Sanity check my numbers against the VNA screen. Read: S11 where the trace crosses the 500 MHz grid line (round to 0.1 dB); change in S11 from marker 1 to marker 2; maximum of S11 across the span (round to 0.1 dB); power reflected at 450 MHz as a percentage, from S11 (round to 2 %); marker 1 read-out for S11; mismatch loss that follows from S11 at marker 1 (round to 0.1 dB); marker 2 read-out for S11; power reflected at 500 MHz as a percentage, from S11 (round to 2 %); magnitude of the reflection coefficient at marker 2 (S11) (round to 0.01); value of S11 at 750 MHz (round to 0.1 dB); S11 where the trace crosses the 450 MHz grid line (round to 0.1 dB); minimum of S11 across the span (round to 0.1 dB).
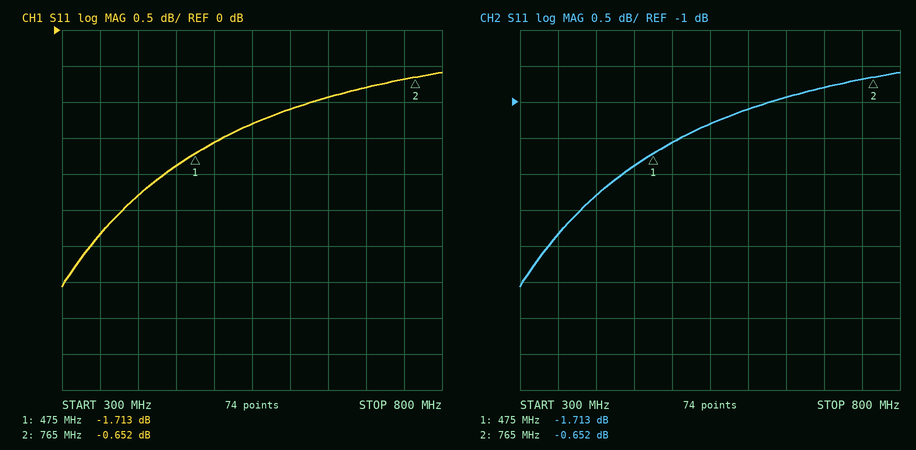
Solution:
-1.6 dB
1.061 dB
-0.6 dB
64 %
-1.713 dB
4.9 dB
-0.652 dB
70 %
0.93
-0.7 dB
-1.9 dB
-3.6 dB
